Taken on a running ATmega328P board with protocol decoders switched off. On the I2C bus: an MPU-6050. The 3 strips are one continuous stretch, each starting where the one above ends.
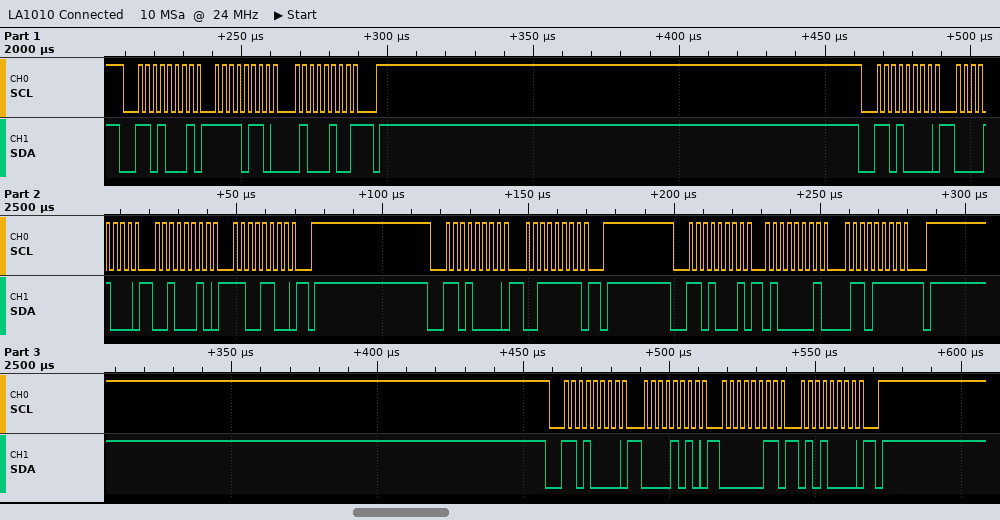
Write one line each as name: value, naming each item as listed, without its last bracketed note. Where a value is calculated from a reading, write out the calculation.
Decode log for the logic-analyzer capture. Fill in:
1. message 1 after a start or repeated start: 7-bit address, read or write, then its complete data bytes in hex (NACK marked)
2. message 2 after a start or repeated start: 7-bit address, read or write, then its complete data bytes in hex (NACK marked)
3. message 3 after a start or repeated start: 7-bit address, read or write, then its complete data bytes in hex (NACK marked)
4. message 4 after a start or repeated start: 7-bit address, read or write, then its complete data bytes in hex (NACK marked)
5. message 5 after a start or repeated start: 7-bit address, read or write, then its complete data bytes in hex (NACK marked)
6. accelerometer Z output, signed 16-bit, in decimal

message 1 after a start or repeated start: 7-bit address, read or write, then its complete data bytes in hex: 0x68 read: F6 44 NACK
message 2 after a start or repeated start: 7-bit address, read or write, then its complete data bytes in hex: 0x68 write: 08 22 CC
message 3 after a start or repeated start: 7-bit address, read or write, then its complete data bytes in hex: 0x68 write: 3F
message 4 after a start or repeated start: 7-bit address, read or write, then its complete data bytes in hex: 0x68 read: 41 6F NACK
message 5 after a start or repeated start: 7-bit address, read or write, then its complete data bytes in hex: 0x68 write: 0A 03 50
accelerometer Z output, signed 16-bit, in decimal: 0x416F = 16751
